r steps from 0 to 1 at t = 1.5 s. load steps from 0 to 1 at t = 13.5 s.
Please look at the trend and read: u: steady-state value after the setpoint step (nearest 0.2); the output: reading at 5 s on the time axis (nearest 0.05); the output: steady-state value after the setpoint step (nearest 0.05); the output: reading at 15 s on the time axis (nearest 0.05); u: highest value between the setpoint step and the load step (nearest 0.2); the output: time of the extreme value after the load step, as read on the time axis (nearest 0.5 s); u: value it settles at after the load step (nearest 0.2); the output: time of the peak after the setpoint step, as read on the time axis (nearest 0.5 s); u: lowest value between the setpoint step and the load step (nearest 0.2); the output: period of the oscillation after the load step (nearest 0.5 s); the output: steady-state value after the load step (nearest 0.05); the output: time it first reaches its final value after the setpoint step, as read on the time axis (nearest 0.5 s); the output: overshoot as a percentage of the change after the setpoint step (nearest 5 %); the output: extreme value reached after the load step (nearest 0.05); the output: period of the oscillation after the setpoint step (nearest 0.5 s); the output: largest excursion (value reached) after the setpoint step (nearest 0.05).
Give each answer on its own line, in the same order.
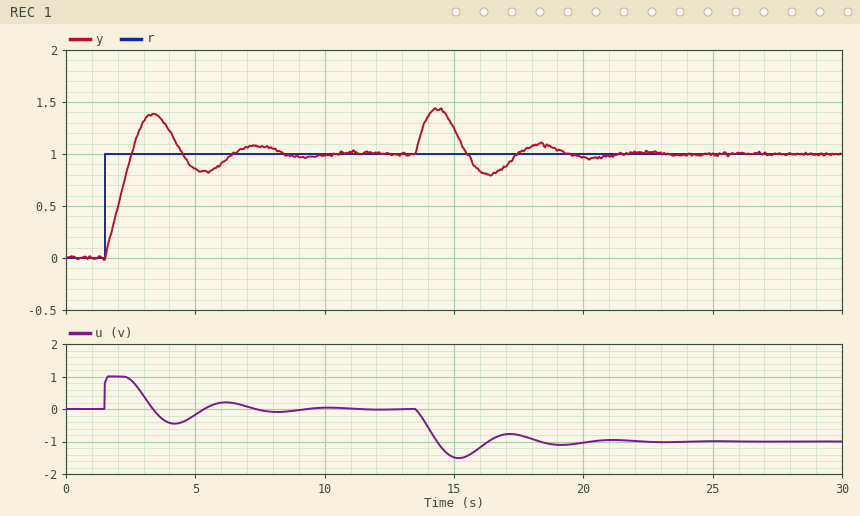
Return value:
0.0
0.85
1.00
1.25
1.0
14.5 s
-1.0
3.5 s
-0.4
4.0 s
1.00
2.5 s
40 %
1.45
4.0 s
1.40
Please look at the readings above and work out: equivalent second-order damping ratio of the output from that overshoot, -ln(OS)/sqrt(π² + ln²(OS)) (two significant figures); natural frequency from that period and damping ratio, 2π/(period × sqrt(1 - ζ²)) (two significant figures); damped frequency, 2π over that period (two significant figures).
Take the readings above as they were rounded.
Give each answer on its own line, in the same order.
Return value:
0.28
1.6 rad/s
1.6 rad/s
